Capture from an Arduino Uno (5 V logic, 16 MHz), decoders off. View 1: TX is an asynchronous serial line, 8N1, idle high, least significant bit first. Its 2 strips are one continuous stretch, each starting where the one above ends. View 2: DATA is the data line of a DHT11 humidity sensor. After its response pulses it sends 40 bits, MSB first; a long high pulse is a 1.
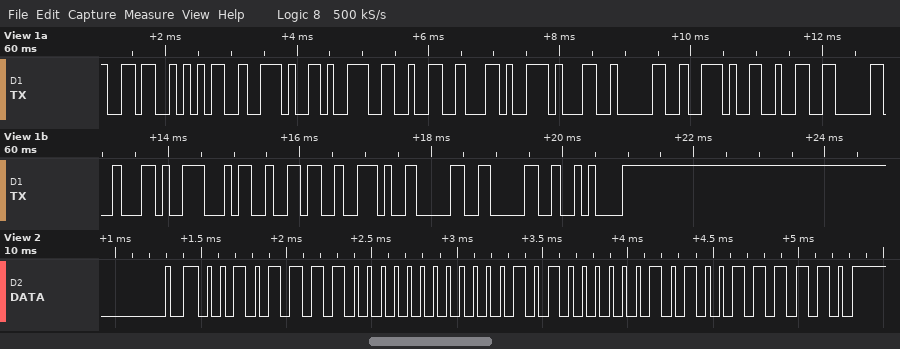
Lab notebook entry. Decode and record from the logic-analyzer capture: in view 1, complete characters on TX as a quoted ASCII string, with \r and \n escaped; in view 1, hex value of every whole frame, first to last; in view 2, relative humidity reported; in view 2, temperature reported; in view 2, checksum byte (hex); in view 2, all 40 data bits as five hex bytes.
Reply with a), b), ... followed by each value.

a) "65.92,10.20,46.00\n"
b) 0x36 0x35 0x2E 0x39 0x32 0x2C 0x31 0x30 0x2E 0x32 0x30 0x2C 0x34 0x36 0x2E 0x30 0x30 0x0A
c) 47 %
d) 10.5 °C
e) 0x3E
f) 2F 00 0A 05 3E
